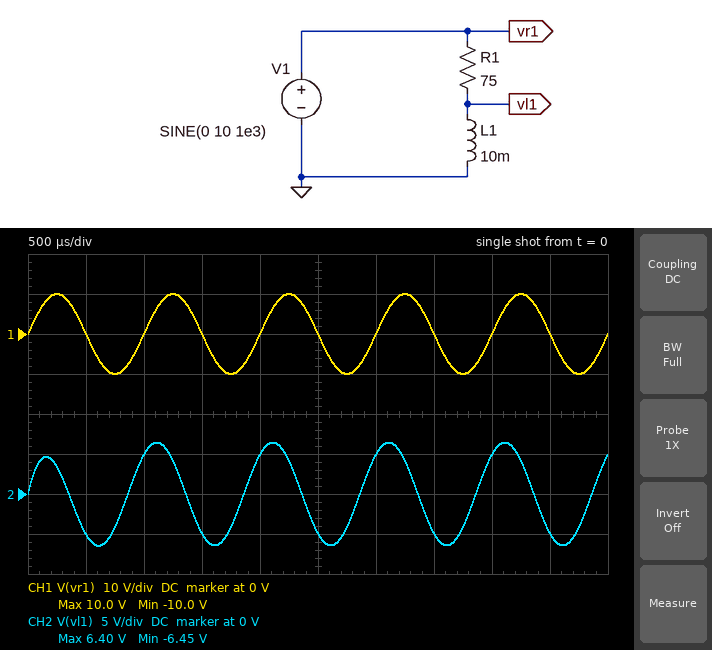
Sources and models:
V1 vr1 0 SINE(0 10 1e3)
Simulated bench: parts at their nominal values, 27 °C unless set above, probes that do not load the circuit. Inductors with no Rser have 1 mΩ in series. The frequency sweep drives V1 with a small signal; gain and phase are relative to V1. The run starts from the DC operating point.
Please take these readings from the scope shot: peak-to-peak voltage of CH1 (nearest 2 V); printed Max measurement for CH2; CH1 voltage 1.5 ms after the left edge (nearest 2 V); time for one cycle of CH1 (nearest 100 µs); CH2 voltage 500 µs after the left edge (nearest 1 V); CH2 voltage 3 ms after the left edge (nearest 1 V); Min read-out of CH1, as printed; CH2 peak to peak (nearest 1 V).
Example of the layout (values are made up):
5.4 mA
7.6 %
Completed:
20 V
6.40 V
0 V
1.0 ms
-5 V
5 V
-10.0 V
13 V
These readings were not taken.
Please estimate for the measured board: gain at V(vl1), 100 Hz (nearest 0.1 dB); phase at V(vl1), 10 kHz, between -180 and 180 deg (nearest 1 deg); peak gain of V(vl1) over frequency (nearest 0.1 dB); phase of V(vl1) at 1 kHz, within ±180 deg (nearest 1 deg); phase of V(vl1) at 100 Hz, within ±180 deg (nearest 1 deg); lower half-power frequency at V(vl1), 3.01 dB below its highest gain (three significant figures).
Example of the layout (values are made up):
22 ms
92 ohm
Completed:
-21.6 dB
7 deg
0 dB
50 deg
85 deg
1.19 kHz
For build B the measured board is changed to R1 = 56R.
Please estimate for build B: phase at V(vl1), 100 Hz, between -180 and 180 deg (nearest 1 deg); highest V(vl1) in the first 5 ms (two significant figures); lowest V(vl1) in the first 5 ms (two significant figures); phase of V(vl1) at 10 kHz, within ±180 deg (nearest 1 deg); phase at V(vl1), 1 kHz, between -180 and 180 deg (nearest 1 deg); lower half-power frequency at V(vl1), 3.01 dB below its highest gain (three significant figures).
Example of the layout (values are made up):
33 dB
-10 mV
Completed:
84 deg
7.5 V
-7.6 V
5 deg
42 deg
891 Hz
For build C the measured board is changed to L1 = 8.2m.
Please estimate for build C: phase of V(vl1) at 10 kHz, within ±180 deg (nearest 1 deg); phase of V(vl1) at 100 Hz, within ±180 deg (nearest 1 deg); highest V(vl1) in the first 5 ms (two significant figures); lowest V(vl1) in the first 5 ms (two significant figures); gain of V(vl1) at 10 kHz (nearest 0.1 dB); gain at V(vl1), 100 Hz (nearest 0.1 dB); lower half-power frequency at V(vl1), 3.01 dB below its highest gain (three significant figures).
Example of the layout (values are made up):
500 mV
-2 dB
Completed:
8 deg
86 deg
5.7 V
-5.7 V
-0.1 dB
-23.3 dB
1.46 kHz
